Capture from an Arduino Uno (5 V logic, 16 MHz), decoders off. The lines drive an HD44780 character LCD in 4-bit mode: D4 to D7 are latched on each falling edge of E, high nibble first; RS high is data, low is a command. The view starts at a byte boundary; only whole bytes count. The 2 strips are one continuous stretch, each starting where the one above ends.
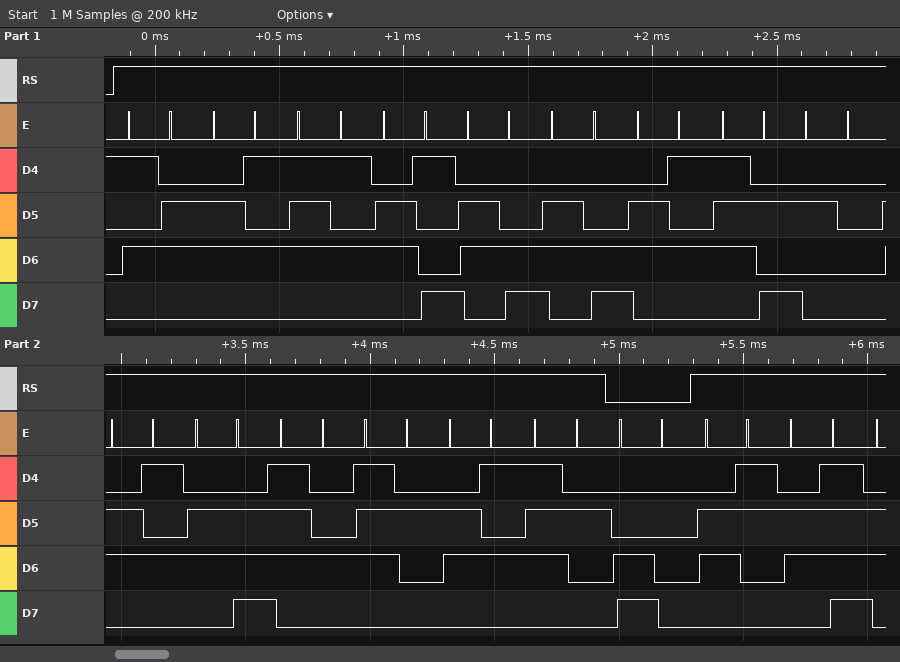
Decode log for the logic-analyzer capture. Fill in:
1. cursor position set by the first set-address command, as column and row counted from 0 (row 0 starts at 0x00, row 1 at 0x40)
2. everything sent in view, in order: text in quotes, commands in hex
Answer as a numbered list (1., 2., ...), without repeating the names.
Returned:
1. column 0, row 1
2. "Veuillez entrer" 0xC0 "co"
